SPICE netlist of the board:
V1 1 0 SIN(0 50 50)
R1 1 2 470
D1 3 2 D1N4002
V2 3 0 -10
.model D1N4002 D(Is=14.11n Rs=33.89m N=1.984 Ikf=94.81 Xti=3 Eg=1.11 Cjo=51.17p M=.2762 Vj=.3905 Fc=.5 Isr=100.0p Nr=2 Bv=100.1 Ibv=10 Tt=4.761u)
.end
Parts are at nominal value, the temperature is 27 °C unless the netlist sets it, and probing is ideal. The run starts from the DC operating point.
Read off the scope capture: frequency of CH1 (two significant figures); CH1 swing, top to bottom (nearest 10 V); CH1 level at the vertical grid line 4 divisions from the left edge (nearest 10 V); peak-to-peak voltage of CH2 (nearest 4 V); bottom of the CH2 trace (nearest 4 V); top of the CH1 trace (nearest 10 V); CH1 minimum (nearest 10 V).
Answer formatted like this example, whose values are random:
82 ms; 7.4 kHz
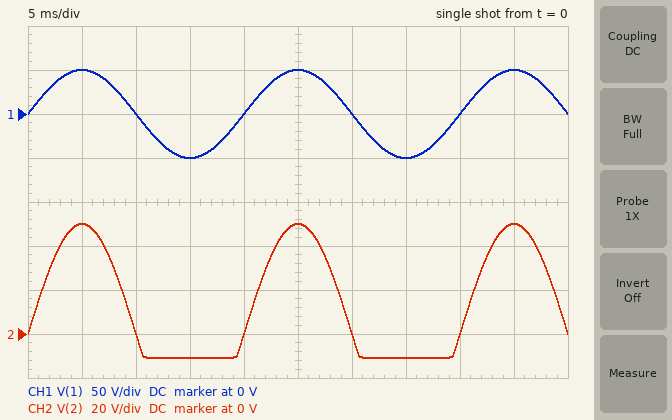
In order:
50 Hz; 100 V; 0 V; 60 V; -12 V; 50 V; -50 V
